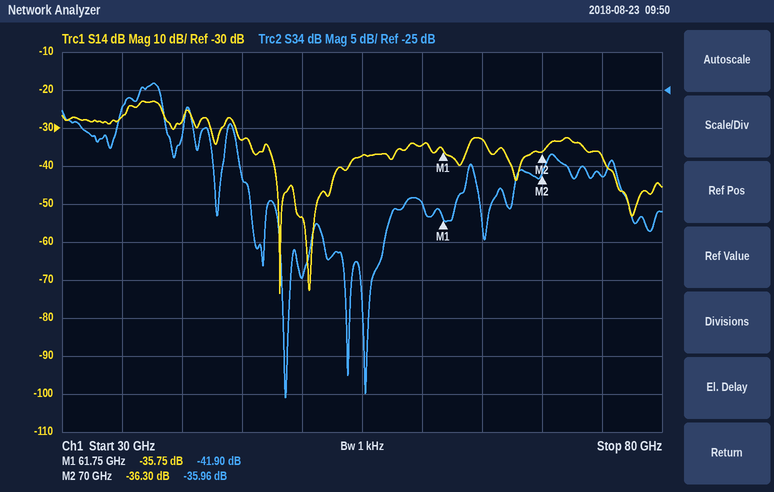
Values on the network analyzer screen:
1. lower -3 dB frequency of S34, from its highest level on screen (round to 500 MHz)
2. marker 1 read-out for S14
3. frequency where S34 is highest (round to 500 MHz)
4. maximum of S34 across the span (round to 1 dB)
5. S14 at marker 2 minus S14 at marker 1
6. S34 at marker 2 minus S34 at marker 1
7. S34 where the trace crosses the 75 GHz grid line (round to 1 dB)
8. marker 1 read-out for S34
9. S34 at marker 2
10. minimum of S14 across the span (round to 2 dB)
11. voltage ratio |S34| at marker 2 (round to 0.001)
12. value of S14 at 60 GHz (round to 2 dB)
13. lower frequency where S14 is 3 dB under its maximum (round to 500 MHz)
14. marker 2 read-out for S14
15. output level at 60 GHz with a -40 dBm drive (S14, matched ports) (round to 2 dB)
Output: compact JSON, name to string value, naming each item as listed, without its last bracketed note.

{"lower -3 dB frequency of S34, from its highest level on screen": "35.0 GHz", "marker 1 read-out for S14": "-35.75 dB", "frequency where S34 is highest": "37.5 GHz", "maximum of S34 across the span": "-24 dB", "S14 at marker 2 minus S14 at marker 1": "-0.55 dB", "S34 at marker 2 minus S34 at marker 1": "5.94 dB", "S34 where the trace crosses the 75 GHz grid line": "-36 dB", "marker 1 read-out for S34": "-41.90 dB", "S34 at marker 2": "-35.96 dB", "minimum of S14 across the span": "-74 dB", "voltage ratio |S34| at marker 2": "0.016", "value of S14 at 60 GHz": "-34 dB", "lower frequency where S14 is 3 dB under its maximum": "35.5 GHz", "marker 2 read-out for S14": "-36.30 dB", "output level at 60 GHz with a -40 dBm drive (S14, matched ports)": "-74 dBm"}
